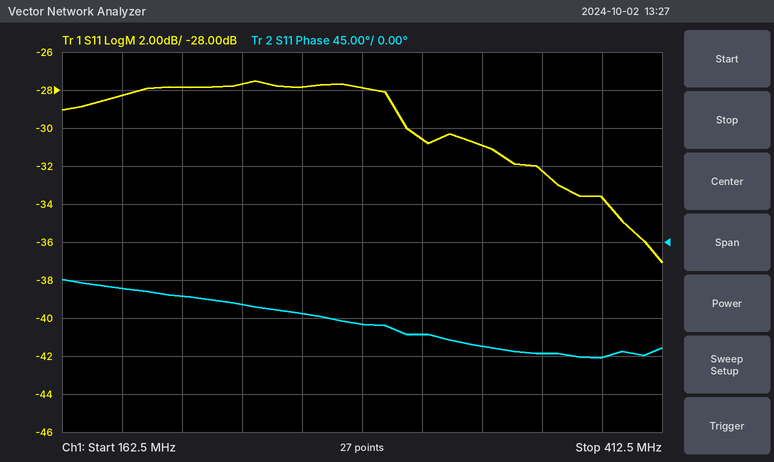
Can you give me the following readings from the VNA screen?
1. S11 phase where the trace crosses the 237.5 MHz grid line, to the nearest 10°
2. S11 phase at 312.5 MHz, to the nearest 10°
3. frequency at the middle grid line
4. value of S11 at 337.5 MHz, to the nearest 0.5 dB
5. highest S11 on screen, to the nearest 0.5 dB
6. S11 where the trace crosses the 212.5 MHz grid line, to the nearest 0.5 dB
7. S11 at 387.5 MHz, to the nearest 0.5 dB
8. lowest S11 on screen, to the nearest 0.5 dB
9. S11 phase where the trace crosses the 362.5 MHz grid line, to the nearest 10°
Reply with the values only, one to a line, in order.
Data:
-70°
-110°
287.5 MHz
-31.0 dB
-27.5 dB
-28.0 dB
-33.5 dB
-37.0 dB
-130°
